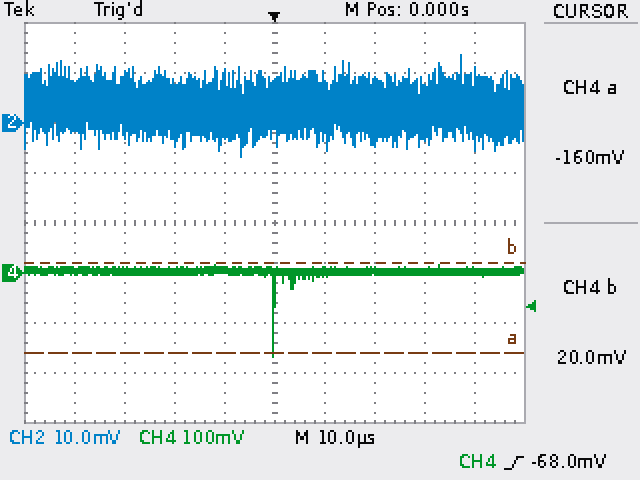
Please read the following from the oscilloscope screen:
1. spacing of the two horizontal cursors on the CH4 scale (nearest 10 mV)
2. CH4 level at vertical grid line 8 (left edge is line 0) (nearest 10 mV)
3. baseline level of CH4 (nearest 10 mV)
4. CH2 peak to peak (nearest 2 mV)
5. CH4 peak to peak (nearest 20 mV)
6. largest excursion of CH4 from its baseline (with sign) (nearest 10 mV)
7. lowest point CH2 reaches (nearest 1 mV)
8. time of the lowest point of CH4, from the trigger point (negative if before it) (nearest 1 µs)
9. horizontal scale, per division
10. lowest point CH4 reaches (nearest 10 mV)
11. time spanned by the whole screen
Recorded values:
180 mV
0 mV
0 mV
20 mV
180 mV
-170 mV
-7 mV
0 µs
10 µs
-170 mV
100 µs
